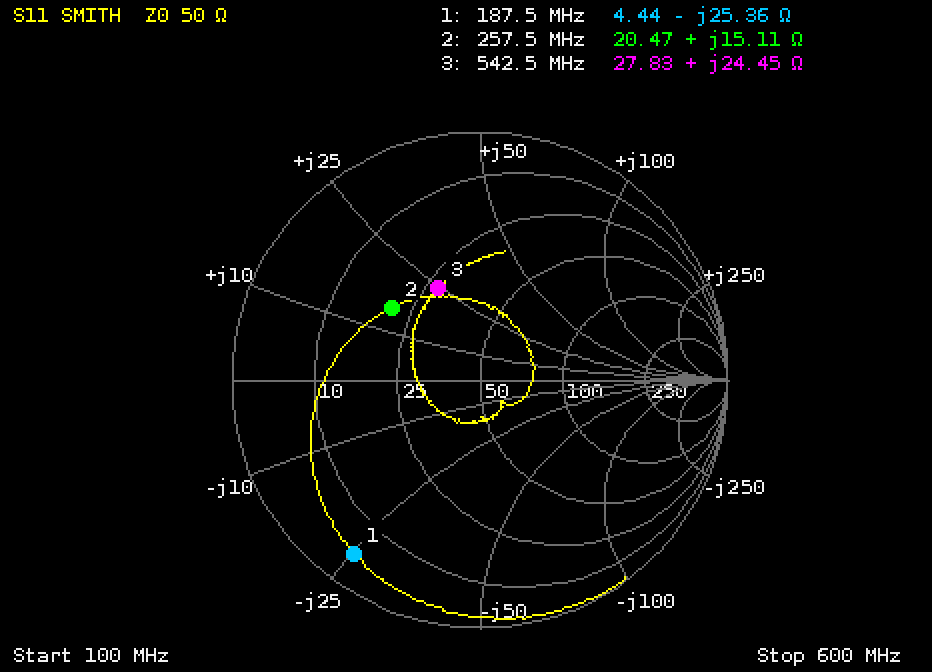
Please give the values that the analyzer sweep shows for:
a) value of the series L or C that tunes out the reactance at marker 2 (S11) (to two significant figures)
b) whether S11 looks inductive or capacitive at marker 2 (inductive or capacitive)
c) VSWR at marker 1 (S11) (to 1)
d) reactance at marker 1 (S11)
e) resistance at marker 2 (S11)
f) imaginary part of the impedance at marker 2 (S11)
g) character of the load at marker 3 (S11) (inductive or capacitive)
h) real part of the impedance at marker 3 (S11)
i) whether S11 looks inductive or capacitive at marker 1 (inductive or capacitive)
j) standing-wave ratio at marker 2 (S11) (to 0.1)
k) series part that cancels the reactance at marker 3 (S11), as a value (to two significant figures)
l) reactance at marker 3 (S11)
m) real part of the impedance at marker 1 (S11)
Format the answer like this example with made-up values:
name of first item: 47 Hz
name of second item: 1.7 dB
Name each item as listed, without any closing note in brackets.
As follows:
value of the series L or C that tunes out the reactance at marker 2 (S11): 41 pF
whether S11 looks inductive or capacitive at marker 2: inductive
VSWR at marker 1 (S11): 14
reactance at marker 1: -25.36 Ω
resistance at marker 2: 20.47 Ω
imaginary part of the impedance at marker 2: +15.11 Ω
character of the load at marker 3 (S11): inductive
real part of the impedance at marker 3: 27.83 Ω
whether S11 looks inductive or capacitive at marker 1: capacitive
standing-wave ratio at marker 2 (S11): 2.7
series part that cancels the reactance at marker 3 (S11), as a value: 12 pF
reactance at marker 3: +24.45 Ω
real part of the impedance at marker 1: 4.44 Ω
